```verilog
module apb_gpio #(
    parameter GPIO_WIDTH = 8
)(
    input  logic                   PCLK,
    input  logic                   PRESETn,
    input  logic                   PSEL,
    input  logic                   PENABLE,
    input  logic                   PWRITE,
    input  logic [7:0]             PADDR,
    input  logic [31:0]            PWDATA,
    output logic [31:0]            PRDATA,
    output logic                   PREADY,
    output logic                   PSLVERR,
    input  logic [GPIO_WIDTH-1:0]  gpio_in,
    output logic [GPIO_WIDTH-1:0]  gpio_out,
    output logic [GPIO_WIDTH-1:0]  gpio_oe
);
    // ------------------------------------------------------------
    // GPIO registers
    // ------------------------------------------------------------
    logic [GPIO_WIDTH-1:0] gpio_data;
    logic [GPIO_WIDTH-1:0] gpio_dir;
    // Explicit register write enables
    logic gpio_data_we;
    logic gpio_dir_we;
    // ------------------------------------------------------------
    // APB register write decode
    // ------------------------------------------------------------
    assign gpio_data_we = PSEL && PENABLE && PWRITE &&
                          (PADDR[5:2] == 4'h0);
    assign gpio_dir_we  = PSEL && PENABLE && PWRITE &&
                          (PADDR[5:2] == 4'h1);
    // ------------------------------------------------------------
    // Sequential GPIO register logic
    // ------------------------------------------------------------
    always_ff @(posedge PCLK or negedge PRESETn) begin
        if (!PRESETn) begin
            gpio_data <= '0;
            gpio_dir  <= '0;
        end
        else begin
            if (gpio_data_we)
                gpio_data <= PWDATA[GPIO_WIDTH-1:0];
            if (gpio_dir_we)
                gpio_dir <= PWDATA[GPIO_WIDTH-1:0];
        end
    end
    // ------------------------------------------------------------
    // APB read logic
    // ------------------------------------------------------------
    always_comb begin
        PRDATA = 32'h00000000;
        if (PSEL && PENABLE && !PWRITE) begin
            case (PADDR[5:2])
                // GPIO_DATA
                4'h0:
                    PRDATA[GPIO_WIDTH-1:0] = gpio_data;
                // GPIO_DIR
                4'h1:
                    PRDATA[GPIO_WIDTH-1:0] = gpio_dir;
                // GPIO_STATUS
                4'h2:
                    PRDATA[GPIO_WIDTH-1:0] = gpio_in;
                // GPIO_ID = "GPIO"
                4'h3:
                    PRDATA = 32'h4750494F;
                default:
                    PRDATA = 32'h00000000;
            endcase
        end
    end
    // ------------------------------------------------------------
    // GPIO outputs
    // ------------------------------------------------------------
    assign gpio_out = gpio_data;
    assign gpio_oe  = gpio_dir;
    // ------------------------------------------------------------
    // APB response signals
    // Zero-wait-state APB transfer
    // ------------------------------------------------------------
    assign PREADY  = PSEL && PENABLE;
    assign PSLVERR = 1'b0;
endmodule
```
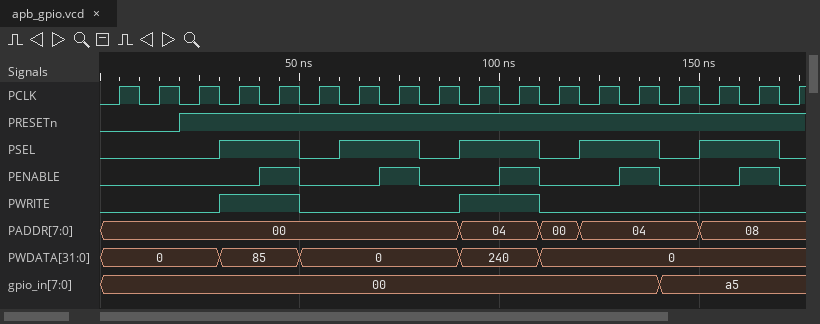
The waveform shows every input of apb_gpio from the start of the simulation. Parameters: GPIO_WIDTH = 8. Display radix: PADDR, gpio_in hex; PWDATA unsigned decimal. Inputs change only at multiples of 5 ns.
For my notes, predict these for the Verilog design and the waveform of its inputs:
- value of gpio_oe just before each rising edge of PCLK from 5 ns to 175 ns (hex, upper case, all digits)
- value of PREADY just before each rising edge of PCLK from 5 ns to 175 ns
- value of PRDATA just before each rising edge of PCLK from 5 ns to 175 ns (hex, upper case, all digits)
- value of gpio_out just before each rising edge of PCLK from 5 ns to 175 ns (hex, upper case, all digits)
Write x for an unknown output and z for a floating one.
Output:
00, 00, 00, 00, 00, 00, 00, 00, 00, 00, 00, F0, F0, F0, F0, F0, F0, F0
0 0 0 0 1 0 0 1 0 0 1 0 0 1 0 0 1 0
00000000, 00000000, 00000000, 00000000, 00000000, 00000000, 00000000, 00000055, 00000000, 00000000, 00000000, 00000000, 00000000, 000000F0, 00000000, 00000000, 000000A5, 00000000
00, 00, 00, 00, 00, 55, 55, 55, 55, 55, 55, 55, 55, 55, 55, 55, 55, 55
